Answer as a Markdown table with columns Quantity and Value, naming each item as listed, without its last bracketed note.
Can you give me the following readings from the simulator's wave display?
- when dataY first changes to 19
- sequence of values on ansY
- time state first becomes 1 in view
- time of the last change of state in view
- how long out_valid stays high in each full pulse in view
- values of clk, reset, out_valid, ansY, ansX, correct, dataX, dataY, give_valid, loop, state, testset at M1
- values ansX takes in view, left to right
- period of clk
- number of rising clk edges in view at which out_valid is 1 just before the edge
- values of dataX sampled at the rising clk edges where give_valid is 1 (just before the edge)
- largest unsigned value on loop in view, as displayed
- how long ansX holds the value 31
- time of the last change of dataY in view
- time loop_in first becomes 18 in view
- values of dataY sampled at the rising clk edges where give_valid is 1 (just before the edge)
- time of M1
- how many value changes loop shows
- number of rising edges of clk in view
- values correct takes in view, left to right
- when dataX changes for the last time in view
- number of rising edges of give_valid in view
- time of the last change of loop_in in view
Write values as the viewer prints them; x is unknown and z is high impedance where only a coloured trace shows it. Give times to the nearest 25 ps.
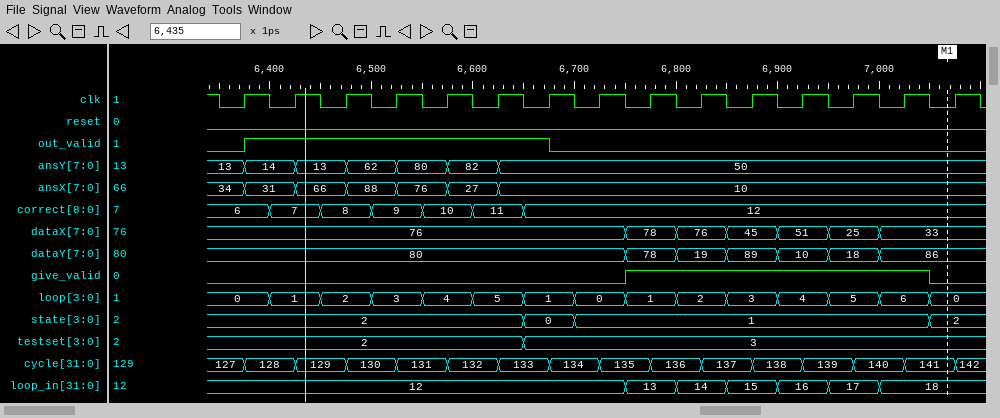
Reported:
| Quantity | Value |
|---|---|
| when dataY first changes to 19 | 6800 ps |
| sequence of values on ansY | 13, 14, 13, 62, 80, 82, 50 |
| time state first becomes 1 in view | 6700 ps |
| time of the last change of state in view | 7050 ps |
| how long out_valid stays high in each full pulse in view | 300 ps |
| values of clk, reset, out_valid, ansY, ansX, correct, dataX, dataY, give_valid, loop, state, testset at M1 | clk=0, reset=0, out_valid=0, ansY=50, ansX=10, correct=12, dataX=33, dataY=86, give_valid=0, loop=0, state=2, testset=3 |
| values ansX takes in view, left to right | 34, 31, 66, 88, 76, 27, 10 |
| period of clk | 50 ps |
| number of rising clk edges in view at which out_valid is 1 just before the edge | 6 |
| values of dataX sampled at the rising clk edges where give_valid is 1 | 78, 76, 45, 51, 25, 33 |
| largest unsigned value on loop in view, as displayed | 6 |
| how long ansX holds the value 31 | 50 ps |
| time of the last change of dataY in view | 7000 ps |
| time loop_in first becomes 18 in view | 7000 ps |
| values of dataY sampled at the rising clk edges where give_valid is 1 | 78, 19, 89, 10, 18, 86 |
| time of M1 | 7075 ps |
| how many value changes loop shows | 14 |
| number of rising edges of clk in view | 15 |
| values correct takes in view, left to right | 6, 7, 8, 9, 10, 11, 12 |
| when dataX changes for the last time in view | 7000 ps |
| number of rising edges of give_valid in view | 1 |
| time of the last change of loop_in in view | 7000 ps |
